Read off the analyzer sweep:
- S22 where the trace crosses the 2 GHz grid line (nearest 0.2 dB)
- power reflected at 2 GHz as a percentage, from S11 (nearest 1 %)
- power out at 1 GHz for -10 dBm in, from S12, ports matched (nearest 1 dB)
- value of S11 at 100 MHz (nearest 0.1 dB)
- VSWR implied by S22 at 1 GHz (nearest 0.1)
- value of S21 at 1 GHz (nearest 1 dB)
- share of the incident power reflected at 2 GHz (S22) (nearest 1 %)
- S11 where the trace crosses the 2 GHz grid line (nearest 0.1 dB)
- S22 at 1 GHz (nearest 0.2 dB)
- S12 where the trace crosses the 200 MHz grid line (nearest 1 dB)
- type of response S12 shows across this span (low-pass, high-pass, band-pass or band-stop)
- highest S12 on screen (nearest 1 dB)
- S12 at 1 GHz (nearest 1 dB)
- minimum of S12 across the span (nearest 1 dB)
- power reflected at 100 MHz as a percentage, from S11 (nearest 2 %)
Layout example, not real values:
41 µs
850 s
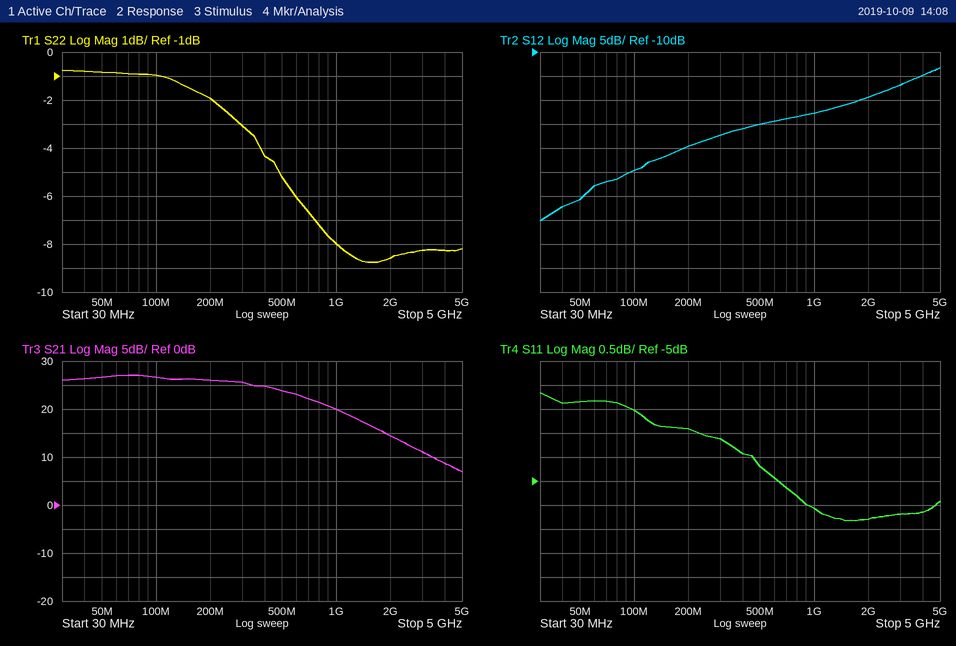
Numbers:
-8.6 dB
26 %
-33 dBm
-3.5 dB
2.3
20 dB
14 %
-5.8 dB
-8.0 dB
-30 dB
high-pass
-13 dB
-23 dB
-45 dB
44 %
